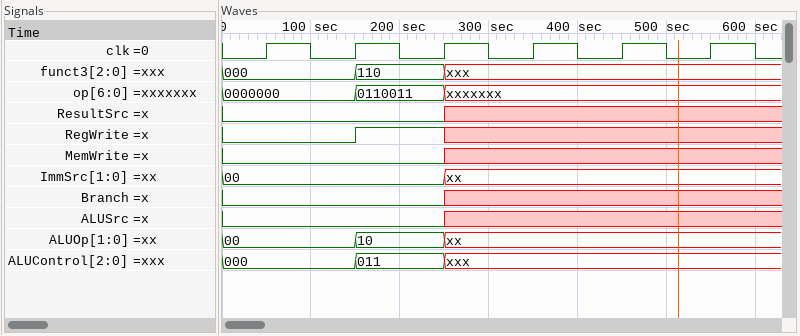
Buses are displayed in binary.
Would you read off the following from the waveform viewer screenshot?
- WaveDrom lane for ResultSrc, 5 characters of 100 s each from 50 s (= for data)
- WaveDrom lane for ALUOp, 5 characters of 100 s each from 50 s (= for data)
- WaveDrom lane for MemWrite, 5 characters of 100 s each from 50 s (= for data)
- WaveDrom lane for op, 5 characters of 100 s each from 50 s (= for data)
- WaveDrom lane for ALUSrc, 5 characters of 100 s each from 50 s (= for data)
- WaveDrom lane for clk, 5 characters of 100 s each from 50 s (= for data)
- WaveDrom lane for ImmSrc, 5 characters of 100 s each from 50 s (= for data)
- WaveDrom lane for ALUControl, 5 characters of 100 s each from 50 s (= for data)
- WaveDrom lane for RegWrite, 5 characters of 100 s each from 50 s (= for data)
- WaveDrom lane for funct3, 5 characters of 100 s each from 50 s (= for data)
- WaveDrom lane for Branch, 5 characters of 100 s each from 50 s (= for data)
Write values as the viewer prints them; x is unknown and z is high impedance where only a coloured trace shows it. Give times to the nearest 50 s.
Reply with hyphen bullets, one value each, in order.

- {name: 'ResultSrc', wave: '0.x..'}
- {name: 'ALUOp', wave: '==x..', data: '00 10'}
- {name: 'MemWrite', wave: '0.x..'}
- {name: 'op', wave: '==x..', data: '0000000 0110011'}
- {name: 'ALUSrc', wave: '0.x..'}
- {name: 'clk', wave: 'p....'}
- {name: 'ImmSrc', wave: '=.x..', data: '00'}
- {name: 'ALUControl', wave: '==x..', data: '000 011'}
- {name: 'RegWrite', wave: '01x..'}
- {name: 'funct3', wave: '==x..', data: '000 110'}
- {name: 'Branch', wave: '0.x..'}
